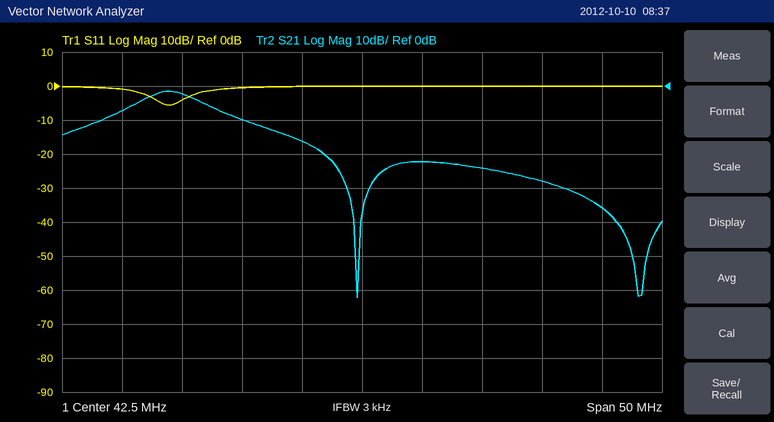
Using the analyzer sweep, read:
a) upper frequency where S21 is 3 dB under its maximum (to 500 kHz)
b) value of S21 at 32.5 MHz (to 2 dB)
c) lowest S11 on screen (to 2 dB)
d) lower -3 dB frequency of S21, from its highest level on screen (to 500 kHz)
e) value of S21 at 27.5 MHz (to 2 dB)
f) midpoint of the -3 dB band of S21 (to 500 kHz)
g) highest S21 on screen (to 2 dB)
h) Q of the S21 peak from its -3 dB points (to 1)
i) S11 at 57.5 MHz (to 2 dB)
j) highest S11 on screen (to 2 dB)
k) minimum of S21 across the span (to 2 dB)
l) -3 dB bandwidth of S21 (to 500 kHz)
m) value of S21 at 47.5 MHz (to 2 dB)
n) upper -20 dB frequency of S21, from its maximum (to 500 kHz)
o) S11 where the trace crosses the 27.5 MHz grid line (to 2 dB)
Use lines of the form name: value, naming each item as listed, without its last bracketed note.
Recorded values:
upper frequency where S21 is 3 dB under its maximum: 29.0 MHz
value of S21 at 32.5 MHz: -10 dB
lowest S11 on screen: -6 dB
lower -3 dB frequency of S21, from its highest level on screen: 24.0 MHz
value of S21 at 27.5 MHz: -2 dB
midpoint of the -3 dB band of S21: 26.5 MHz
highest S21 on screen: -2 dB
Q of the S21 peak from its -3 dB points: 5
S11 at 57.5 MHz: 0 dB
highest S11 on screen: 0 dB
minimum of S21 across the span: -62 dB
-3 dB bandwidth of S21: 5.0 MHz
value of S21 at 47.5 MHz: -22 dB
upper -20 dB frequency of S21, from its maximum: 40.0 MHz
S11 where the trace crosses the 27.5 MHz grid line: -4 dB
